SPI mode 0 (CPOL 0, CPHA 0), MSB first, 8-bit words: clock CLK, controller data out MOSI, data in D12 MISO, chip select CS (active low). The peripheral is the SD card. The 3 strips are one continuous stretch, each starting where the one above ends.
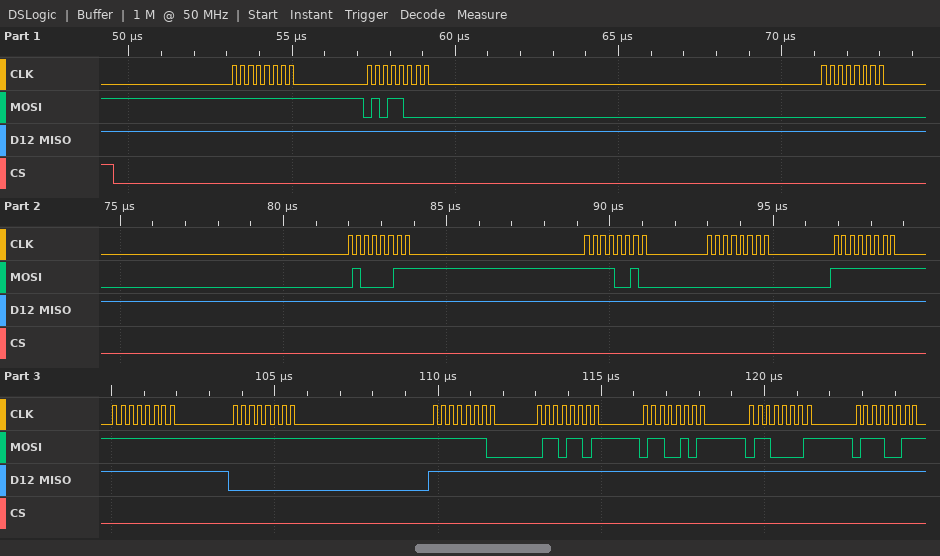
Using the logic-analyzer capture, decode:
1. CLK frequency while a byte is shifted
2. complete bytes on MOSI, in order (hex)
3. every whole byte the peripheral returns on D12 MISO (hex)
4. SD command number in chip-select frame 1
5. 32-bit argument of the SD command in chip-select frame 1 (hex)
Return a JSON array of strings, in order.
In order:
["4 MHz", "0xFF 0x58 0x00 0x43 0xF2 0x00 0xFF 0xFF 0xFF 0xFE 0x6D 0x65 0x61 0x73", "0xFF 0xFF 0xFF 0xFF 0xFF 0xFF 0xFF 0xFF 0x00 0xFF 0xFF 0xFF 0xFF 0xFF", "CMD24", "0x0043F200"]
